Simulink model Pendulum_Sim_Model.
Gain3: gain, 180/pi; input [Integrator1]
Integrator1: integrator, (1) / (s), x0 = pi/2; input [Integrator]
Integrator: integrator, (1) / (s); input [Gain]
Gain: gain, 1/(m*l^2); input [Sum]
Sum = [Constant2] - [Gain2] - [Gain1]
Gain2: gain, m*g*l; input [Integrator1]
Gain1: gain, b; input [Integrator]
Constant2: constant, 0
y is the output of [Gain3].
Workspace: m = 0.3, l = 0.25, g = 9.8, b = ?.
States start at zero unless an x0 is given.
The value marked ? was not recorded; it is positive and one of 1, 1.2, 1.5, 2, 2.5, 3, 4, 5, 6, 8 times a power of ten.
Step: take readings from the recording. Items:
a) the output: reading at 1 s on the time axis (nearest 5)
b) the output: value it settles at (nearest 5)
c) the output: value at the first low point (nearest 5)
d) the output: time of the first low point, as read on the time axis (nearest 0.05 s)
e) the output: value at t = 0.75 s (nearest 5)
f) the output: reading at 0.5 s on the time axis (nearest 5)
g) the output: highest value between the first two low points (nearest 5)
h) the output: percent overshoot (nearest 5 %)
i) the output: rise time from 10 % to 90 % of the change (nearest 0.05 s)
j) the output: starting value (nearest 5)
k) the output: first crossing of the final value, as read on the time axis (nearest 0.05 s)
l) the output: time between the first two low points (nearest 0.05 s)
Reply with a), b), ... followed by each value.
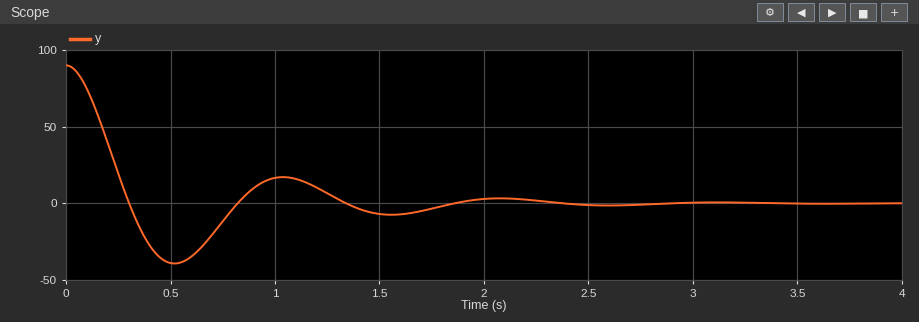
a) 15
b) 0
c) -40
d) 0.50 s
e) -10
f) -40
g) 15
h) 45 %
i) 0.20 s
j) 90
k) 0.30 s
l) 1.05 s
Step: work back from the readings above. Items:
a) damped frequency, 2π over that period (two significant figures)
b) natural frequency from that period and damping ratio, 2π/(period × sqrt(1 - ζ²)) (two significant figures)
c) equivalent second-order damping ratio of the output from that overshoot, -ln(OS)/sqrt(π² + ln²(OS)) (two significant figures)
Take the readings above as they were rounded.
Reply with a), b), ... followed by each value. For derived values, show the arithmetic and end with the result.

a) 2π / 1.05 = 6.0 rad/s
b) 2π / (1.05 × sqrt(1 - 0.25²)) = 6.2 rad/s
c) ln(0.45) = -0.799; 0.799 / sqrt(9.870 + 0.638) = 0.25
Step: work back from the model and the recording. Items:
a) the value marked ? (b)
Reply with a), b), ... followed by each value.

a) 0.06
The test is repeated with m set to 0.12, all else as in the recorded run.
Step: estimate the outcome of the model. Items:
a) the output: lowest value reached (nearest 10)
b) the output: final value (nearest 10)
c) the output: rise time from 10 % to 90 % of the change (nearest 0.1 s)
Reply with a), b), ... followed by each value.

a) -10
b) 0
c) 0.3 s
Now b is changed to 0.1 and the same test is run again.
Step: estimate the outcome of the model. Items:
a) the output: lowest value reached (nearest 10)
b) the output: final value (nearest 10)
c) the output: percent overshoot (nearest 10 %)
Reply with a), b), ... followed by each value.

a) -20
b) 0
c) 20 %
